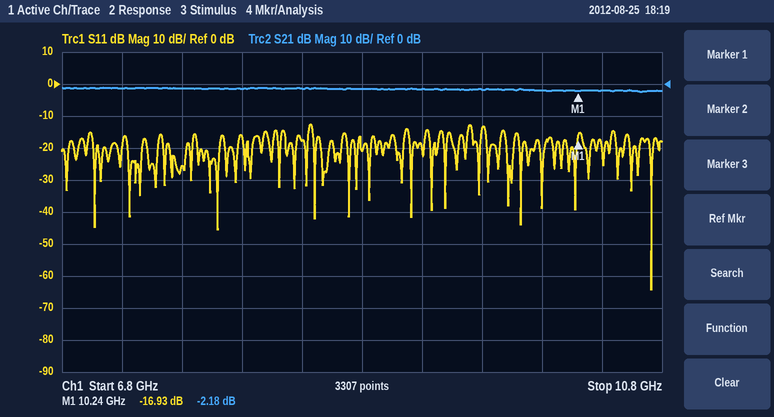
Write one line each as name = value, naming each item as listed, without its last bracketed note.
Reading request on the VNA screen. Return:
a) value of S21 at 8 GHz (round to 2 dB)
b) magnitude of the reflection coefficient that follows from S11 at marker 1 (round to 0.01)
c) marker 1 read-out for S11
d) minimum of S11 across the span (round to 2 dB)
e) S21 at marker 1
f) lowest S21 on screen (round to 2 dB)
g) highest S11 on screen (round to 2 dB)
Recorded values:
value of S21 at 8 GHz = -2 dB
magnitude of the reflection coefficient that follows from S11 at marker 1 = 0.14
marker 1 read-out for S11 = -16.93 dB
minimum of S11 across the span = -64 dB
S21 at marker 1 = -2.18 dB
lowest S21 on screen = -2 dB
highest S11 on screen = -12 dB
